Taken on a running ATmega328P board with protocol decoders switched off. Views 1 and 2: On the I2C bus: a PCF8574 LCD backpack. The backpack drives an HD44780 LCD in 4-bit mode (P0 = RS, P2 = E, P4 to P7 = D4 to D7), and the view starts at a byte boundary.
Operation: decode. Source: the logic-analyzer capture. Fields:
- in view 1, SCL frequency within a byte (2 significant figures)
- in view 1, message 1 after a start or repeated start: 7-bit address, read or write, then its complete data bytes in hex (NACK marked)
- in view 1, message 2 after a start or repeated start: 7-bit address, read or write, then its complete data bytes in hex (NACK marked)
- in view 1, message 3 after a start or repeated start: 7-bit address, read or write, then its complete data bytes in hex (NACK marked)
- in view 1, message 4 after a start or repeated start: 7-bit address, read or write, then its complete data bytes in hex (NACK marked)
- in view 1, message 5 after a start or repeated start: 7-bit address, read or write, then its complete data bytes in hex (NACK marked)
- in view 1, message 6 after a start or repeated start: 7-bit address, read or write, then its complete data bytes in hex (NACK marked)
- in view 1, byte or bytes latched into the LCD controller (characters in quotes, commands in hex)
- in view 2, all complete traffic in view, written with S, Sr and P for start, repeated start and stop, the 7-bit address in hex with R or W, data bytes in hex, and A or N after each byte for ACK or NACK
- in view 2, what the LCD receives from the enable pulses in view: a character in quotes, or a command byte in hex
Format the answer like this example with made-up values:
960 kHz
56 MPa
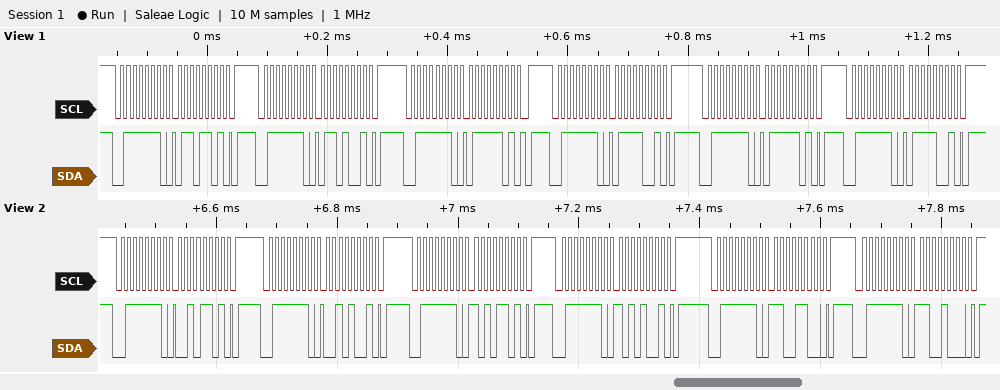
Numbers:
100 kHz
0x3F write: 6D
0x3F write: 69
0x3F write: 7D
0x3F write: 79
0x3F write: 7D
0x3F write: 79
'g'
S 3FW A 2D A P S 3FW A 29 A P S 3FW A AD A P S 3FW A A9 A P S 3FW A CC A P S 3FW A C8 A P
'*'
